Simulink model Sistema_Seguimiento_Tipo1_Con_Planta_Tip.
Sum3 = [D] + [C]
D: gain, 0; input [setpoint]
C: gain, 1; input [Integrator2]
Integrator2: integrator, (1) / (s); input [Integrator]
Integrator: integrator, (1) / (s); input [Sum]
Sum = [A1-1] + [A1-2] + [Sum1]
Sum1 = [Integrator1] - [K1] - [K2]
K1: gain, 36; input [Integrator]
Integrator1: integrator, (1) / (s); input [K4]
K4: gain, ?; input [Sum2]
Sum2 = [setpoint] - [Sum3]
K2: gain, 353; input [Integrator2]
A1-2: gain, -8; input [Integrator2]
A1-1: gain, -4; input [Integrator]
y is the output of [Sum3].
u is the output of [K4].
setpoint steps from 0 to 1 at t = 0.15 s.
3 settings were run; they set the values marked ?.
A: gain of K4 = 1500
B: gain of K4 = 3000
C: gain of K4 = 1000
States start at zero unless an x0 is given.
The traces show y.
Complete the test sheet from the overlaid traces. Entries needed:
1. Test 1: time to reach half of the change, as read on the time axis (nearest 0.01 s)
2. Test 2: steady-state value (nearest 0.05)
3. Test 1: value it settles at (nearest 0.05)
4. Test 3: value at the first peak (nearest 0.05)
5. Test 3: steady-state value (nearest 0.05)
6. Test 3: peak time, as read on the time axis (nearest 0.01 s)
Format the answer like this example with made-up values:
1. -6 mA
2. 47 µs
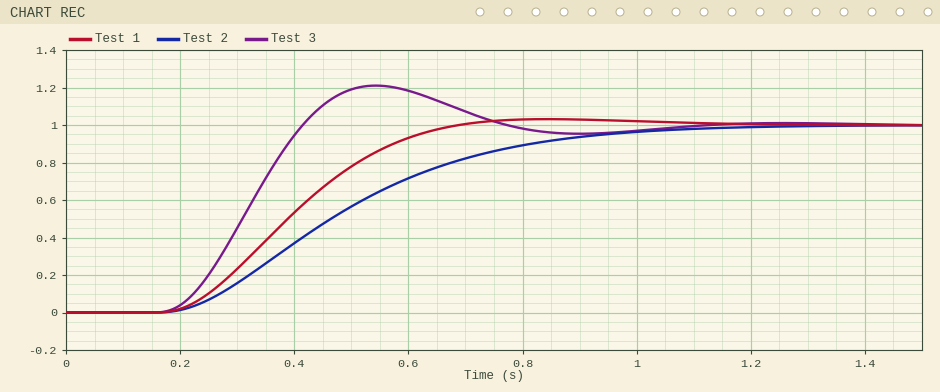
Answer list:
1. 0.39 s
2. 1.00
3. 1.00
4. 1.20
5. 1.00
6. 0.54 s
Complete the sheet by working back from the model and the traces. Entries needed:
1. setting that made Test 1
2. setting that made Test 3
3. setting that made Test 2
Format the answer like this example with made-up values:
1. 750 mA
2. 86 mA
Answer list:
1. A
2. B
3. C
